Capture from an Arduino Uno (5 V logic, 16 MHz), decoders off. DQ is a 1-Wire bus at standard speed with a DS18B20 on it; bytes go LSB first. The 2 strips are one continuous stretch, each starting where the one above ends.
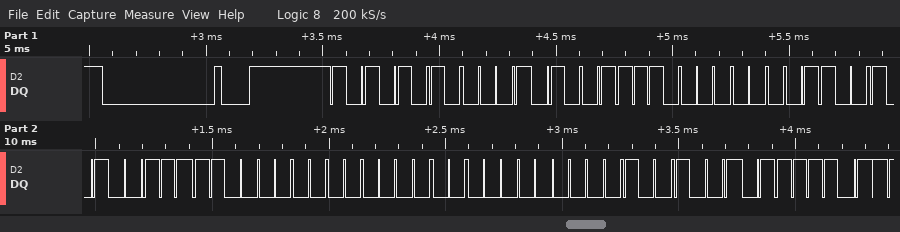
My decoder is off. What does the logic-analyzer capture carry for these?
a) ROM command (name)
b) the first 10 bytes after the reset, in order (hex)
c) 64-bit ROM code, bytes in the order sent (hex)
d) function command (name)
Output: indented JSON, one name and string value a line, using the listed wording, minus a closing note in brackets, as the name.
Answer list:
{
  "ROM command": "Match ROM",
  "the first 10 bytes after the reset, in order": "55 28 0F 30 E5 03 00 00 92 BE",
  "64-bit ROM code, bytes in the order sent": "28 0F 30 E5 03 00 00 92",
  "function command": "Read Scratchpad"
}
